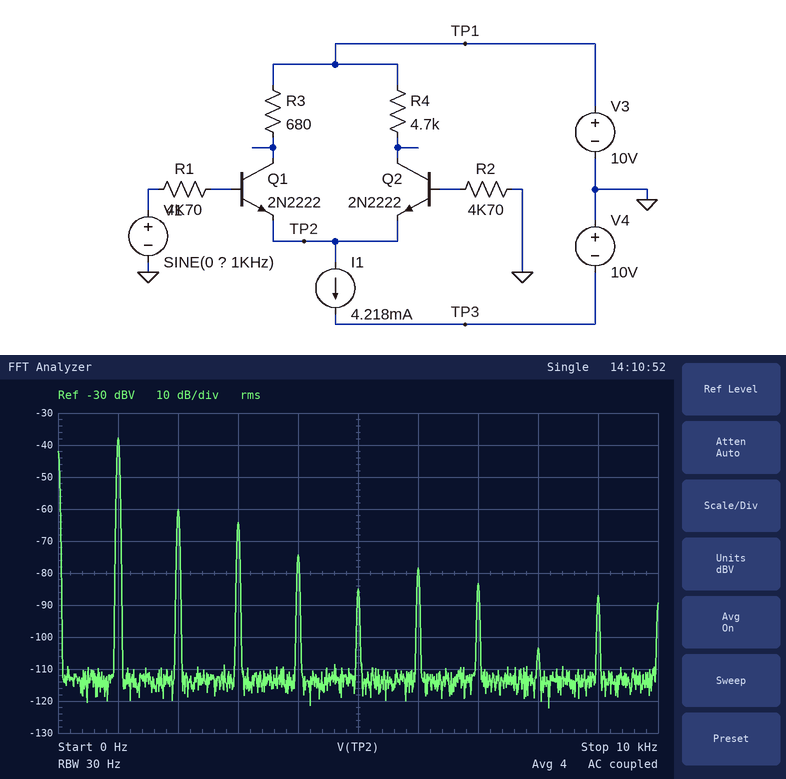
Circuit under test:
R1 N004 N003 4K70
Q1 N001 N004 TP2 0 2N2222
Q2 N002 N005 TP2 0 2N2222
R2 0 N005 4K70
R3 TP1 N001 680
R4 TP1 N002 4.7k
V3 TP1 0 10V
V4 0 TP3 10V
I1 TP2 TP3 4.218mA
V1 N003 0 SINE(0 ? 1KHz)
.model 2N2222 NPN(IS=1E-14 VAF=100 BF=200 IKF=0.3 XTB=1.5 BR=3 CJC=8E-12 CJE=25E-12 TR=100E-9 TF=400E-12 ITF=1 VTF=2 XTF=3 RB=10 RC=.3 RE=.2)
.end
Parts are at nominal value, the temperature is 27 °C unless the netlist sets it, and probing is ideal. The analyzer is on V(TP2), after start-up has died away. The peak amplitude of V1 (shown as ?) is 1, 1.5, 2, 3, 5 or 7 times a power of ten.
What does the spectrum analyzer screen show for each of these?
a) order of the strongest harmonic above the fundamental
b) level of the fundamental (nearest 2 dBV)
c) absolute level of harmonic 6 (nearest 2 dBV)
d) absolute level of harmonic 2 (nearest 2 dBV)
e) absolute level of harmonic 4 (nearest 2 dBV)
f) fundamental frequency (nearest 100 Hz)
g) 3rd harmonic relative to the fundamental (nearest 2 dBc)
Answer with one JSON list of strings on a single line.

["2", "-38 dBV", "-78 dBV", "-60 dBV", "-74 dBV", "1.0 kHz", "-26 dBc"]
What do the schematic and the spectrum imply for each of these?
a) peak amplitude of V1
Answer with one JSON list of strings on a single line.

["30 mV"]
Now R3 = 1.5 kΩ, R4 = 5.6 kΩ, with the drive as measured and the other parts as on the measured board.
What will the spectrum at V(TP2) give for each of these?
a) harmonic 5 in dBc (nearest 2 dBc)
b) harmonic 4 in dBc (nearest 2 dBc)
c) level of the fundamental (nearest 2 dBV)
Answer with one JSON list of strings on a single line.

["-38 dBc", "-46 dBc", "-34 dBV"]
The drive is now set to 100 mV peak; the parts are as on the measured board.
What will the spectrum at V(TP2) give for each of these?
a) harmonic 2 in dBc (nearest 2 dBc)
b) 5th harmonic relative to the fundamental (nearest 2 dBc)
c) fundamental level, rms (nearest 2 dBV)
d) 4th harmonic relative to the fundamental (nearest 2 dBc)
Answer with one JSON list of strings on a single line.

["-20 dBc", "-38 dBc", "-26 dBV", "-34 dBc"]
